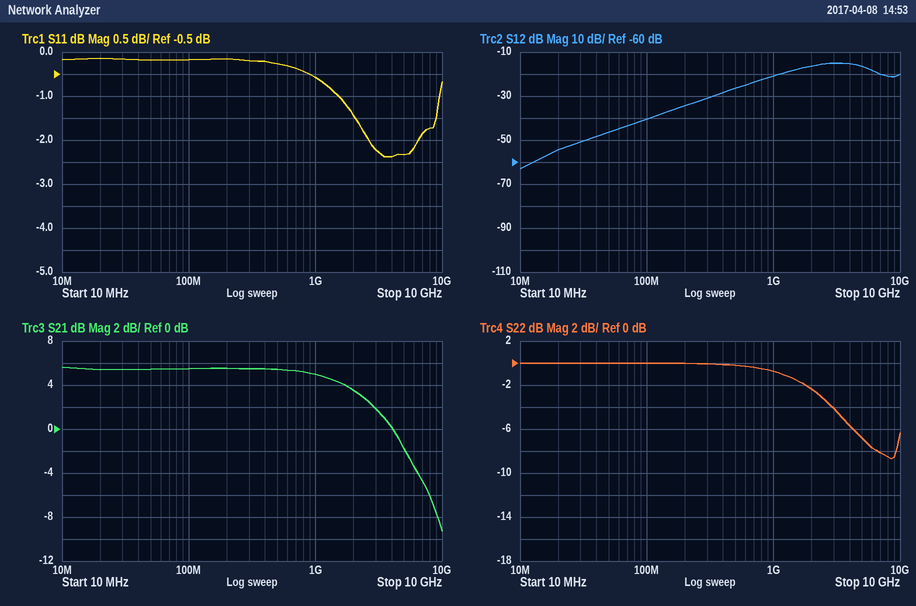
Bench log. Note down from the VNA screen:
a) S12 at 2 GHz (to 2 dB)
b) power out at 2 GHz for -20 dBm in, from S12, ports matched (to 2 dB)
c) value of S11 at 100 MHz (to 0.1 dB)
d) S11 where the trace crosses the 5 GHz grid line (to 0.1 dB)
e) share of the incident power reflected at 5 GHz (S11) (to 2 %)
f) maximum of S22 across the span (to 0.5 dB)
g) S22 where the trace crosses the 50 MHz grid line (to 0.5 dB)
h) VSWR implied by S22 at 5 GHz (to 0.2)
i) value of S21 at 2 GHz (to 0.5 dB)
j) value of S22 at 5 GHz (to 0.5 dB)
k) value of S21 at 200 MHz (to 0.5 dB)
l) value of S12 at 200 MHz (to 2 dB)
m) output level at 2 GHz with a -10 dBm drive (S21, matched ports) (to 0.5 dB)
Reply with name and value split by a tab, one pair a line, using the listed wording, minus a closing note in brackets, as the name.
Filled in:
S12 at 2 GHz	-16 dB
power out at 2 GHz for -20 dBm in, from S12, ports matched	-36 dBm
value of S11 at 100 MHz	-0.2 dB
S11 where the trace crosses the 5 GHz grid line	-2.3 dB
share of the incident power reflected at 5 GHz (S11)	58 %
maximum of S22 across the span	0.0 dB
S22 where the trace crosses the 50 MHz grid line	0.0 dB
VSWR implied by S22 at 5 GHz	2.6
value of S21 at 2 GHz	3.5 dB
value of S22 at 5 GHz	-7.0 dB
value of S21 at 200 MHz	5.5 dB
value of S12 at 200 MHz	-34 dB
output level at 2 GHz with a -10 dBm drive (S21, matched ports)	-6.5 dBm
